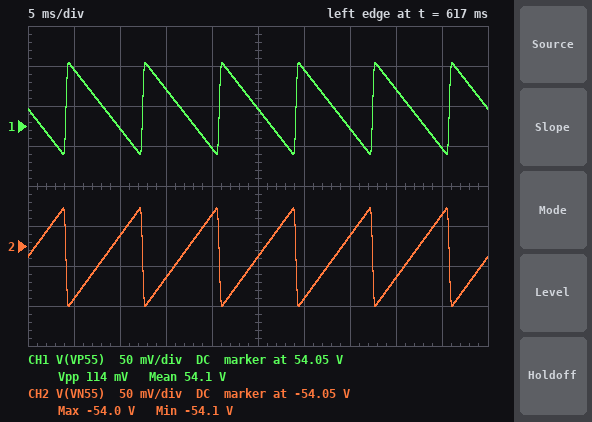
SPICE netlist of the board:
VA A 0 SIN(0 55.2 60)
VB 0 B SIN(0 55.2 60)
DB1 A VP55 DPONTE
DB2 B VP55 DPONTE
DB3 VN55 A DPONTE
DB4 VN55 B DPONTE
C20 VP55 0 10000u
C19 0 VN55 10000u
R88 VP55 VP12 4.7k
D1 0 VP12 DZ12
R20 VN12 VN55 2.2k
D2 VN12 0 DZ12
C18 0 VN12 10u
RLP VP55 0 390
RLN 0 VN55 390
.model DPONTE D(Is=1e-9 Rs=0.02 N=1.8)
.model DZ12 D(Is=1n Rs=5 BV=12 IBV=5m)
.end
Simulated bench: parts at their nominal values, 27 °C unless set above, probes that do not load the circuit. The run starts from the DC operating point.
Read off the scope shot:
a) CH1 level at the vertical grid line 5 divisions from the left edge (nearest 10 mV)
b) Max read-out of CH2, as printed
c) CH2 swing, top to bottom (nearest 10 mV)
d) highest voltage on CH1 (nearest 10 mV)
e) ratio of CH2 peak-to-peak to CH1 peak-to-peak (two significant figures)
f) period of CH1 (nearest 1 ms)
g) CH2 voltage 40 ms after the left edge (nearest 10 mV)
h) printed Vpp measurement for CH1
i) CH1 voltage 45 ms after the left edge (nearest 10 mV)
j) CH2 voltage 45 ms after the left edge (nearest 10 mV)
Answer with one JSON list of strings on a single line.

["54.07 V", "-54.0 V", "120 mV", "54.13 V", "1.1", "8 ms", "-54.09 V", "114 mV", "54.02 V", "-54.01 V"]
